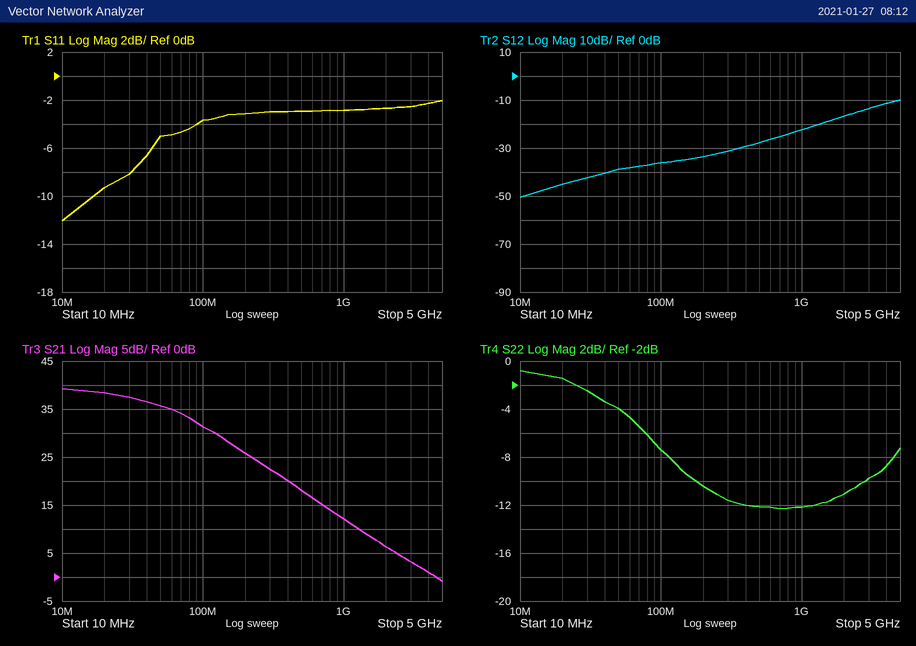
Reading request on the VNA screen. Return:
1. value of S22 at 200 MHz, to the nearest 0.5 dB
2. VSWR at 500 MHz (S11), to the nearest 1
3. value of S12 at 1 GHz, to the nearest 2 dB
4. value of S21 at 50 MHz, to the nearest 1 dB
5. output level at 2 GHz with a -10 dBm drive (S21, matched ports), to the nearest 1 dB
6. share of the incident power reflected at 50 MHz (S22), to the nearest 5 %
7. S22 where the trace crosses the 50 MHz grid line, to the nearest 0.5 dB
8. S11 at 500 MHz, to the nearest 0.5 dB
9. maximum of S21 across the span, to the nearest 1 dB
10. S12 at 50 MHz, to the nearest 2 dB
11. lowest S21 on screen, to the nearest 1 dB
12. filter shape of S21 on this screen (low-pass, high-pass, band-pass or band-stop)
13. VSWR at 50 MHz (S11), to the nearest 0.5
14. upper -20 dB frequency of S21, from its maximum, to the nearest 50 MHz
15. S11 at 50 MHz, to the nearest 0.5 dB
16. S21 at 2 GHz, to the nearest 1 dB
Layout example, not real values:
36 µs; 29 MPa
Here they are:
-10.5 dB; 6; -22 dB; 36 dB; -4 dBm; 40 %; -4.0 dB; -3.0 dB; 39 dB; -38 dB; -1 dB; low-pass; 3.5; 450 MHz; -5.0 dB; 6 dB
